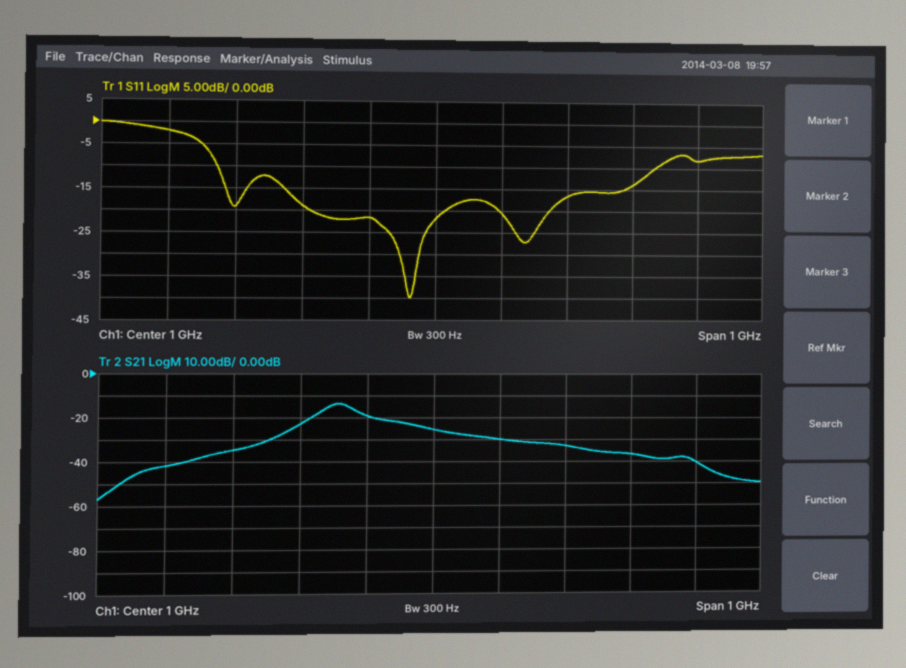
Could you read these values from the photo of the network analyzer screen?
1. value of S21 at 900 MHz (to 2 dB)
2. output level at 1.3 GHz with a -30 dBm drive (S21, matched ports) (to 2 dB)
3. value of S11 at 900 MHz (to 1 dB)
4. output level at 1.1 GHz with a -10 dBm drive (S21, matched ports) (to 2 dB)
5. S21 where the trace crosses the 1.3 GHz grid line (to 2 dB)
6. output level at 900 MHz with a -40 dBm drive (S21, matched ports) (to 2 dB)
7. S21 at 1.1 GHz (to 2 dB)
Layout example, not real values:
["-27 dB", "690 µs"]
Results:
["-20 dB", "-66 dBm", "-22 dB", "-40 dBm", "-36 dB", "-60 dBm", "-30 dB"]
